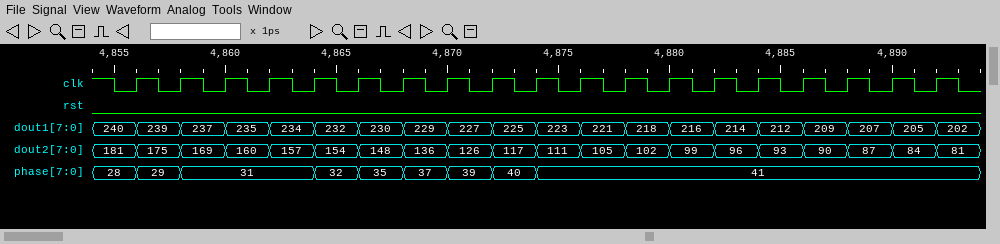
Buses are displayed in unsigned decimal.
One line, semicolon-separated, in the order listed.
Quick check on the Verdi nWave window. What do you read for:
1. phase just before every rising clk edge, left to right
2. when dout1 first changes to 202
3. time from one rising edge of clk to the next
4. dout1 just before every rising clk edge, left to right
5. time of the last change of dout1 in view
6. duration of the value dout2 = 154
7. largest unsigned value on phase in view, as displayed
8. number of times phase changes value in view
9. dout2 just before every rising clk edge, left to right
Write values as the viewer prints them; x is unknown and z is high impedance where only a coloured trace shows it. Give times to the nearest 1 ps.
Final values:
28, 29, 31, 31, 31, 32, 35, 37, 39, 40, 41, 41, 41, 41, 41, 41, 41, 41, 41; 4892 ps; 2 ps; 240, 239, 237, 235, 234, 232, 230, 229, 227, 225, 223, 221, 218, 216, 214, 212, 209, 207, 205; 4892 ps; 2 ps; 41; 8; 181, 175, 169, 160, 157, 154, 148, 136, 126, 117, 111, 105, 102, 99, 96, 93, 90, 87, 84
